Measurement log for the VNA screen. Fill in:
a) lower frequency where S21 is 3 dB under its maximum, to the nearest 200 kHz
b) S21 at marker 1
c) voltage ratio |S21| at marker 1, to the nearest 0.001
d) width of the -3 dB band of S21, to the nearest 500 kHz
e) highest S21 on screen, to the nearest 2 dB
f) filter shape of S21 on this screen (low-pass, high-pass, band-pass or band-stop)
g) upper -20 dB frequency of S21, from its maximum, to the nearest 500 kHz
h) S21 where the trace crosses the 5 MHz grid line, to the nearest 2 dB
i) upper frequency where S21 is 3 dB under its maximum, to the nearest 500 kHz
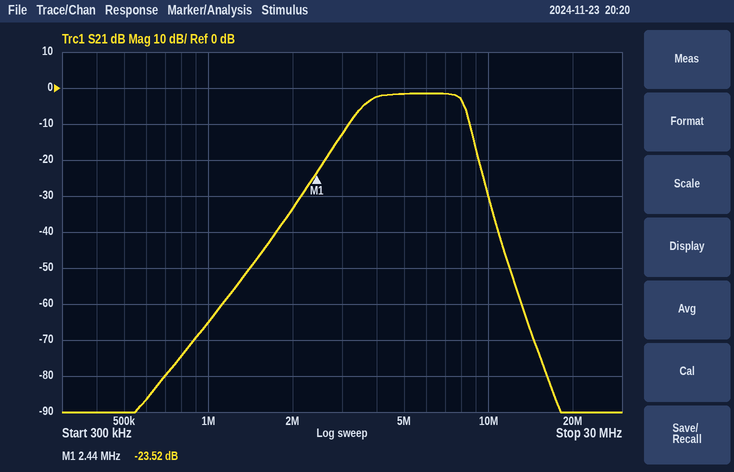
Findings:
3.6 MHz
-23.52 dB
0.067
4.5 MHz
-2 dB
band-pass
9.5 MHz
-2 dB
8.0 MHz
